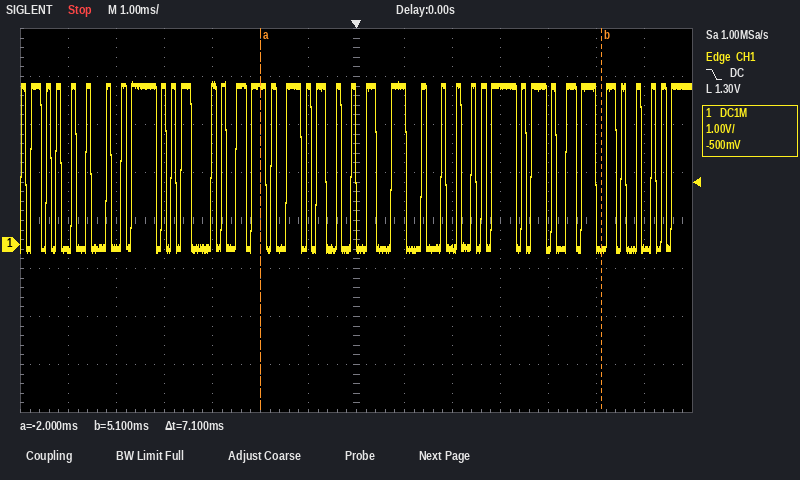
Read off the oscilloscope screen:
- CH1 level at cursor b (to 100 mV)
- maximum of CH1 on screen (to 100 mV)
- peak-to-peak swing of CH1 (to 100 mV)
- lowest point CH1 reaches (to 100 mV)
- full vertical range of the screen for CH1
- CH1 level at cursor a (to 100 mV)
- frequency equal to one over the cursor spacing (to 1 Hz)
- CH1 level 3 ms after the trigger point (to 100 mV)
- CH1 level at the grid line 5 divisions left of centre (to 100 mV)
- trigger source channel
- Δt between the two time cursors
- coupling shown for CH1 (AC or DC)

-100 mV
3.4 V
3.6 V
-200 mV
8 V
3.3 V
141 Hz
3.3 V
-100 mV
CH1
7.1 ms
DC
